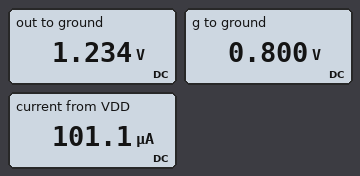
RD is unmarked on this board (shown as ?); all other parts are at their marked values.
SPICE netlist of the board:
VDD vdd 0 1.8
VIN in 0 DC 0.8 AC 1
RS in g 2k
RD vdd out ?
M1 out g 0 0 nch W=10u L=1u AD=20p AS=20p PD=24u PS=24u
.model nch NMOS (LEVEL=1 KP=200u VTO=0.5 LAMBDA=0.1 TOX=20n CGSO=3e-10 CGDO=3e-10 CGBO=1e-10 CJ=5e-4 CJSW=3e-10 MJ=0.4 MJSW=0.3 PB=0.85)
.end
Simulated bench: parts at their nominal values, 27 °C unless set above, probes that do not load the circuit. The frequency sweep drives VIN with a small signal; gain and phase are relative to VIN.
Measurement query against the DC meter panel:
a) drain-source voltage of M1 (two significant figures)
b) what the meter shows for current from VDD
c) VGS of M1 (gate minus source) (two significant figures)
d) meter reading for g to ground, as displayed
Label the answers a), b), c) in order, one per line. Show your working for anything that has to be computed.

a) 1.234 V = 1.2 V
b) 101.1 µA
c) 800 mV = 800 mV
d) 0.800 V
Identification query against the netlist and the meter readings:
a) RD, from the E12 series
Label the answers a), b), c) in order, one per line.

a) 5.6 kΩ
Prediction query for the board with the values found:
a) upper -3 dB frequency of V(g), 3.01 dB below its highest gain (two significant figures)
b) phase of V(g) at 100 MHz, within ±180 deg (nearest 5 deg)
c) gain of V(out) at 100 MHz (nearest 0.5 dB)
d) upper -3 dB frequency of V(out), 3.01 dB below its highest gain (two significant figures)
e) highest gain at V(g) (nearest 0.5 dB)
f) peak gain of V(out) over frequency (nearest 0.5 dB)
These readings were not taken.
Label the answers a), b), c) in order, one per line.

a) 3.0 GHz
b) 0 deg
c) 11.0 dB
d) 1.3 GHz
e) 0 dB
f) 11.0 dB
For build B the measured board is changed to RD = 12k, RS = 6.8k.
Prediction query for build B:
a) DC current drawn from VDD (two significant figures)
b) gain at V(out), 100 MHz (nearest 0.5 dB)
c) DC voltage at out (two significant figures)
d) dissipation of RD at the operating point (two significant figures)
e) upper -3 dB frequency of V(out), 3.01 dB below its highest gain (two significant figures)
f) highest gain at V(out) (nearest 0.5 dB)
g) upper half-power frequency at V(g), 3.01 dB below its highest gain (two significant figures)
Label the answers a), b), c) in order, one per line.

a) 96 µA
b) 16.5 dB
c) 650 mV
d) 110 µW
e) 400 MHz
f) 17.0 dB
g) 520 MHz
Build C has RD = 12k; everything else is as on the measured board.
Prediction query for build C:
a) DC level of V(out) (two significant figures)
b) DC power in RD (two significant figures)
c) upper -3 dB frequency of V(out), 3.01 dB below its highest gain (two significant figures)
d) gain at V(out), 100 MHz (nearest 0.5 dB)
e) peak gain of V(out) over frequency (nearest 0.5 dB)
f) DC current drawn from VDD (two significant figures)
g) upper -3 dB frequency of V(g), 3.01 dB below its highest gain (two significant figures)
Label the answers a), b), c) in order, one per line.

a) 650 mV
b) 110 µW
c) 670 MHz
d) 16.5 dB
e) 17.0 dB
f) 96 µA
g) 3.1 GHz
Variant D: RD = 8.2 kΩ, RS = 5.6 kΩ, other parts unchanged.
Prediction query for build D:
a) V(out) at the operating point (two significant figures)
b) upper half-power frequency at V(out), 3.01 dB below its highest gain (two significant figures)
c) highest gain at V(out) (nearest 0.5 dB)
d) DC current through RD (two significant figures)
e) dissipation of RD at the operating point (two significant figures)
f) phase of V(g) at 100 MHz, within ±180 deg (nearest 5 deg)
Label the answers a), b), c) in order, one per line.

a) 990 mV
b) 590 MHz
c) 14.0 dB
d) 99 µA
e) 80 µW
f) -5 deg
